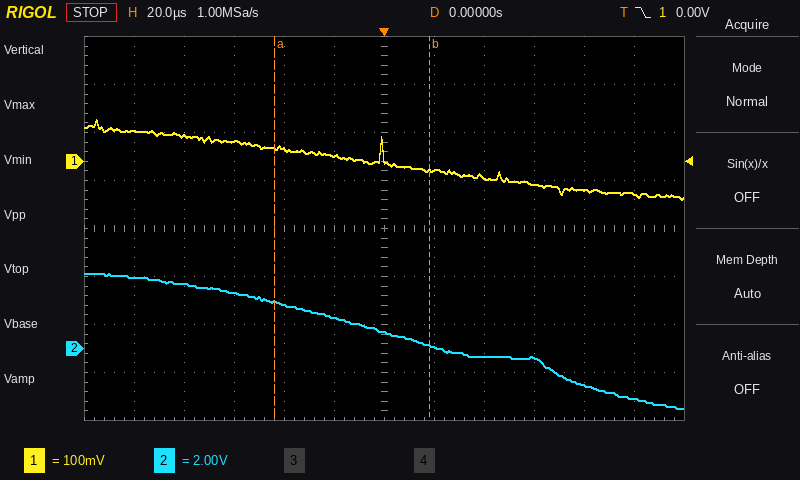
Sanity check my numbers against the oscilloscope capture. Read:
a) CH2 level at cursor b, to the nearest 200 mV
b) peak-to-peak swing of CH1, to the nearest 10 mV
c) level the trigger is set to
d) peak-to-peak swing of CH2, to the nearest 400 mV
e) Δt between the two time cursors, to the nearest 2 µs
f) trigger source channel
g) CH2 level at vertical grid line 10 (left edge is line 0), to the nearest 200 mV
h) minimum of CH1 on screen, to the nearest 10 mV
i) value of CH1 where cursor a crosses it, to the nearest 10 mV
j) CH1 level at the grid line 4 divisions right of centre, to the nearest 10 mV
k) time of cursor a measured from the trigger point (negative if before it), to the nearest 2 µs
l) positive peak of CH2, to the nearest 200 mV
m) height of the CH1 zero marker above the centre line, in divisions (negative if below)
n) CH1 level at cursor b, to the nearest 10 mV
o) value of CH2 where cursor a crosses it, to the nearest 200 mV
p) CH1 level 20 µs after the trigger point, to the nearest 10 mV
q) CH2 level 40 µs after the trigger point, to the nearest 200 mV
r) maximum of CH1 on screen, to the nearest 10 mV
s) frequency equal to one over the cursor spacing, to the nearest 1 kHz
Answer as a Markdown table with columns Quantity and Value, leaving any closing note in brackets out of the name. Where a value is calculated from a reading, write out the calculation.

| Quantity | Value |
|---|---|
| CH2 level at cursor b, to the nearest 200 mV | 200 mV |
| peak-to-peak swing of CH1, to the nearest 10 mV | 90 mV − (-80 mV) = 170 mV |
| level the trigger is set to | 0.00 V |
| peak-to-peak swing of CH2, to the nearest 400 mV | 5.6 V |
| Δt between the two time cursors, to the nearest 2 µs | 62 µs |
| trigger source channel | CH1 |
| CH2 level at vertical grid line 10 (left edge is line 0), to the nearest 200 mV | -1.6 V |
| minimum of CH1 on screen, to the nearest 10 mV | -80 mV |
| value of CH1 where cursor a crosses it, to the nearest 10 mV | 30 mV |
| CH1 level at the grid line 4 divisions right of centre, to the nearest 10 mV | -60 mV |
| time of cursor a measured from the trigger point (negative if before it), to the nearest 2 µs | -44 µs |
| positive peak of CH2, to the nearest 200 mV | 3.2 V |
| height of the CH1 zero marker above the centre line, in divisions | +1.4 div |
| CH1 level at cursor b, to the nearest 10 mV | -20 mV |
| value of CH2 where cursor a crosses it, to the nearest 200 mV | 2.0 V |
| CH1 level 20 µs after the trigger point, to the nearest 10 mV | -20 mV |
| CH2 level 40 µs after the trigger point, to the nearest 200 mV | -400 mV |
| maximum of CH1 on screen, to the nearest 10 mV | 90 mV |
| frequency equal to one over the cursor spacing, to the nearest 1 kHz | 1 / 62 µs ≈ 16 kHz |
